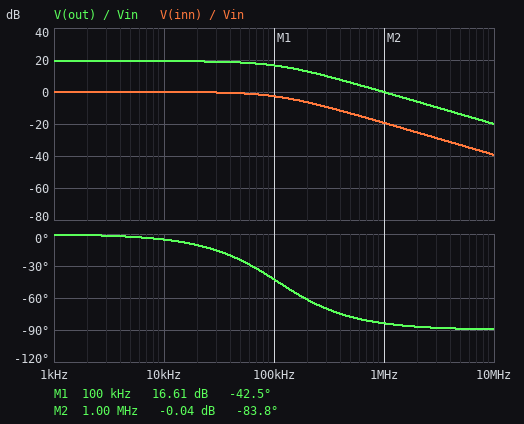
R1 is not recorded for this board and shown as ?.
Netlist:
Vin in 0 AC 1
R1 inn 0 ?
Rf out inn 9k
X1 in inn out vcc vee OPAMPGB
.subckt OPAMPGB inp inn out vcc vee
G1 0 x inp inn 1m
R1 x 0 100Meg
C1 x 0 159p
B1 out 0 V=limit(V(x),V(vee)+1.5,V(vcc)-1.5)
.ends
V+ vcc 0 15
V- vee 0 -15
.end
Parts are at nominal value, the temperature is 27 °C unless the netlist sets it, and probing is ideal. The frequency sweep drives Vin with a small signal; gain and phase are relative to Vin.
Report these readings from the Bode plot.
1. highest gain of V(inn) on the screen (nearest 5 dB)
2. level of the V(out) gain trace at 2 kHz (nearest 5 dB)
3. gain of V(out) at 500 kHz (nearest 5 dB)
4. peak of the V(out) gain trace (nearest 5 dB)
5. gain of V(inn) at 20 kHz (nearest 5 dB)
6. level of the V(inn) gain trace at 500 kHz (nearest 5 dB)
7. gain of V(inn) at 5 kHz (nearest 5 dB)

0 dB
20 dB
5 dB
20 dB
0 dB
-15 dB
0 dB
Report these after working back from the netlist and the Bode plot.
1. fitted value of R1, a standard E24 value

1.1 kΩ
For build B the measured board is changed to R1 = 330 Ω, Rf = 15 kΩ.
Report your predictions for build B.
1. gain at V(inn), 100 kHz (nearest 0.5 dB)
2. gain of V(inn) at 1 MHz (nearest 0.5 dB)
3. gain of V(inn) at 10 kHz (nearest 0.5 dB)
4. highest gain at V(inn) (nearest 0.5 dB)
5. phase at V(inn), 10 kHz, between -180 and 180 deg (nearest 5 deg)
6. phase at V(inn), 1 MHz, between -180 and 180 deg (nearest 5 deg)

-13.5 dB
-33.5 dB
-1.0 dB
0 dB
-25 deg
-90 deg
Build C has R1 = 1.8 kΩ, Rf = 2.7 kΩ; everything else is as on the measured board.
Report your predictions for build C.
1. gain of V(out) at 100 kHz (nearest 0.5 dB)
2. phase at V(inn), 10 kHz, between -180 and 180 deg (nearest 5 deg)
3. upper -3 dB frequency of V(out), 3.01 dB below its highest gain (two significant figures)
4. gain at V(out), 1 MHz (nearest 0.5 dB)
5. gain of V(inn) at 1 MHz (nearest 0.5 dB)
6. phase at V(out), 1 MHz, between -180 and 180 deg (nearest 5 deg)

7.5 dB
0 deg
400 kHz
-0.5 dB
-8.5 dB
-70 deg
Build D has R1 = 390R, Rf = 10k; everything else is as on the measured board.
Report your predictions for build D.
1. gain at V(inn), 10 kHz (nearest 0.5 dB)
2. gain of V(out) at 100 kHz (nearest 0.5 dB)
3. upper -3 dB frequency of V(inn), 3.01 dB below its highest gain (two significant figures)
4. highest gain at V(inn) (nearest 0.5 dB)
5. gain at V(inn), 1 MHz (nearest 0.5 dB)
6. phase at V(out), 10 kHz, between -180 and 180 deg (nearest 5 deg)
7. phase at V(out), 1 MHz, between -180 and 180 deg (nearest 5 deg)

-0.5 dB
19.5 dB
38 kHz
0 dB
-28.5 dB
-15 deg
-90 deg
